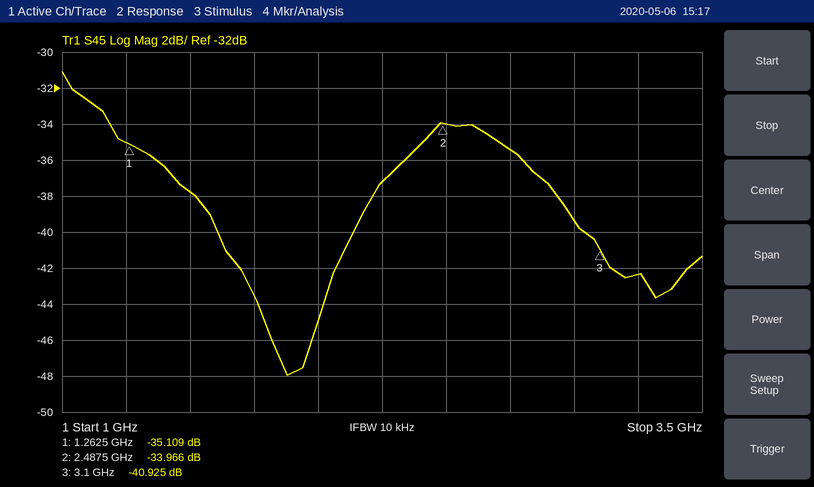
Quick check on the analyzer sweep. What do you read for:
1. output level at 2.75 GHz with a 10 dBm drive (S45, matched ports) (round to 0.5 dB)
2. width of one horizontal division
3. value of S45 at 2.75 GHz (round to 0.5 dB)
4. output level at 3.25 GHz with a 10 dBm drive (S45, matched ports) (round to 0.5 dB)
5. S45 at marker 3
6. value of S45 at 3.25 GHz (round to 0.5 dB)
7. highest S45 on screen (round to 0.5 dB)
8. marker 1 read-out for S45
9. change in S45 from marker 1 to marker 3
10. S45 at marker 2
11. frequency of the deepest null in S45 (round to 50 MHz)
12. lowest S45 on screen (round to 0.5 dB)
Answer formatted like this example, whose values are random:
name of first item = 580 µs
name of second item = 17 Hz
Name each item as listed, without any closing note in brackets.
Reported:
output level at 2.75 GHz with a 10 dBm drive (S45, matched ports) = -25.5 dBm
width of one horizontal division = 250 MHz
value of S45 at 2.75 GHz = -35.5 dB
output level at 3.25 GHz with a 10 dBm drive (S45, matched ports) = -32.5 dBm
S45 at marker 3 = -40.925 dB
value of S45 at 3.25 GHz = -42.5 dB
highest S45 on screen = -31.0 dB
marker 1 read-out for S45 = -35.109 dB
change in S45 from marker 1 to marker 3 = -5.816 dB
S45 at marker 2 = -33.966 dB
frequency of the deepest null in S45 = 1.90 GHz
lowest S45 on screen = -48.0 dB
